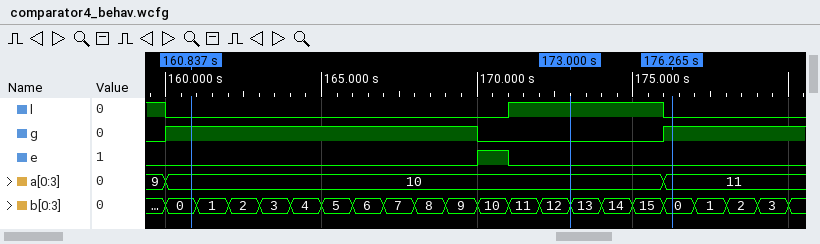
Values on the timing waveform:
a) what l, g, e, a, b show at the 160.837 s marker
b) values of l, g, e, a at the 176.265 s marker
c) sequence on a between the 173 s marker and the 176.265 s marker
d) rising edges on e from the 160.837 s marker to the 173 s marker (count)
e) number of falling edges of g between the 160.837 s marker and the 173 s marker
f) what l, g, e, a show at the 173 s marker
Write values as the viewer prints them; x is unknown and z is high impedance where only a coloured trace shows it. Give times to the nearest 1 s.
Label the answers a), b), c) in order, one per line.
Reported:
a) l=0, g=1, e=0, a=10, b=0
b) l=0, g=1, e=0, a=11
c) 10, 11
d) 1
e) 1
f) l=1, g=0, e=0, a=10
